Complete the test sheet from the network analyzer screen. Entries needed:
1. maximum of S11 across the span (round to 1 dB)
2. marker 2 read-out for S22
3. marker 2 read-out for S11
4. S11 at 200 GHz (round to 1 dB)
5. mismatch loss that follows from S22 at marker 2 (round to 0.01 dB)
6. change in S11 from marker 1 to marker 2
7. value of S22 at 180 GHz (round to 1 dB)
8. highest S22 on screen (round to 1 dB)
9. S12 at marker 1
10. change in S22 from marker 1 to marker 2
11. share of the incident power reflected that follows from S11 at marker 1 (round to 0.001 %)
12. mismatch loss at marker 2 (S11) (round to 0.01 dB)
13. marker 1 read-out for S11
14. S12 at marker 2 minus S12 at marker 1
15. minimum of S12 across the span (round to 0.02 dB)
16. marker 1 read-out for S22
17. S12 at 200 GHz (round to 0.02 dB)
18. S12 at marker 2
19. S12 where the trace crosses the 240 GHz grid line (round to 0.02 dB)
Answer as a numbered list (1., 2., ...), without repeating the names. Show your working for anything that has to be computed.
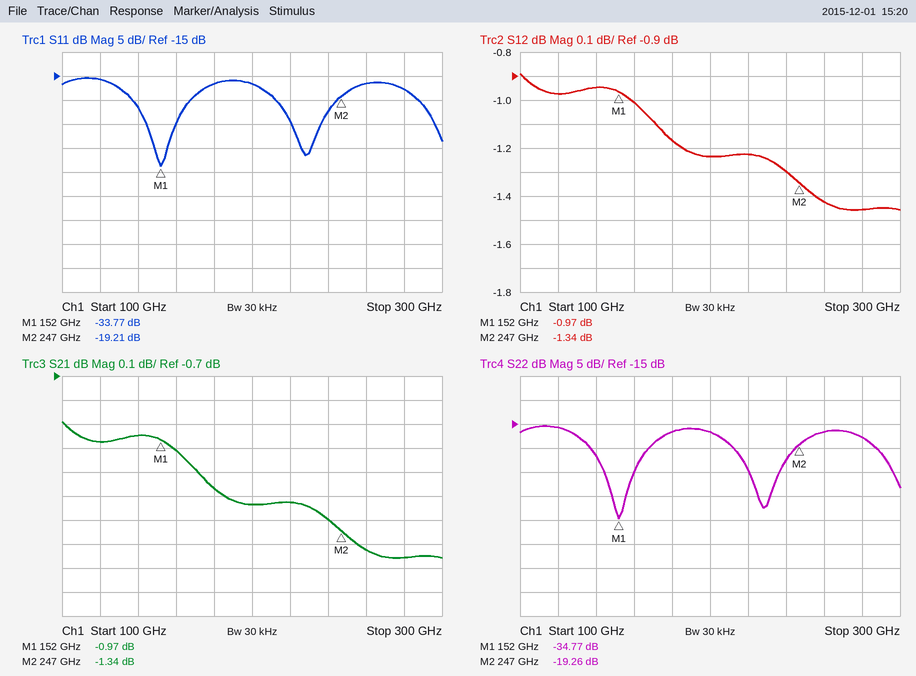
1. -15 dB
2. -19.26 dB
3. -19.21 dB
4. -17 dB
5. −10 log10(1 − 10^(-19.26/10)) ≈ 0.05 dB
6. -19.21 − (-33.77) = 14.56 dB
7. -17 dB
8. -15 dB
9. -0.97 dB
10. -19.26 − (-34.77) = 15.51 dB
11. 10^(-33.77/10) ≈ 0.042 %
12. −10 log10(1 − 10^(-19.21/10)) ≈ 0.05 dB
13. -33.77 dB
14. -1.34 − (-0.97) = -0.37 dB
15. -1.46 dB
16. -34.77 dB
17. -1.24 dB
18. -1.34 dB
19. -1.30 dB
